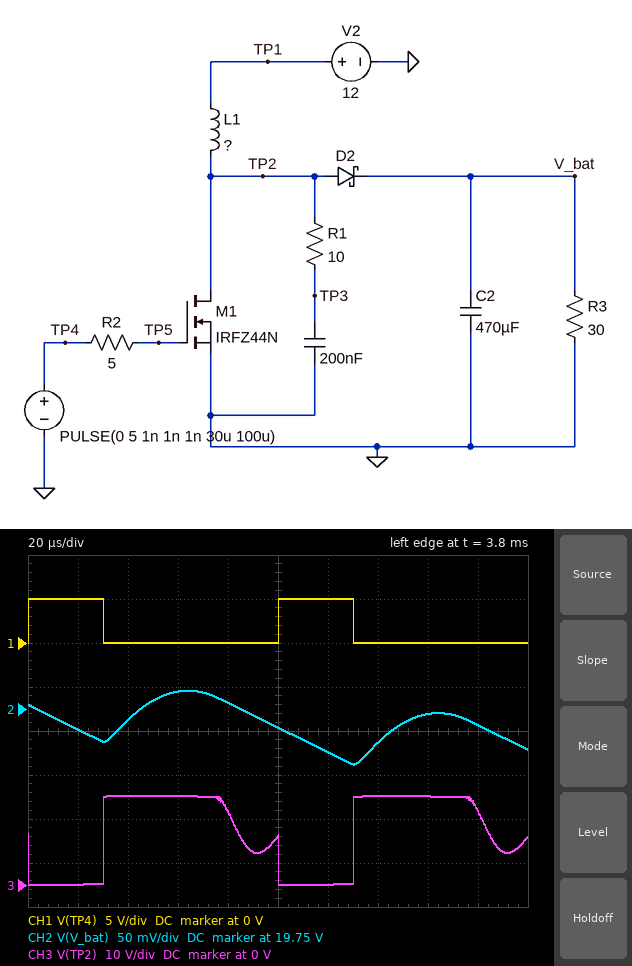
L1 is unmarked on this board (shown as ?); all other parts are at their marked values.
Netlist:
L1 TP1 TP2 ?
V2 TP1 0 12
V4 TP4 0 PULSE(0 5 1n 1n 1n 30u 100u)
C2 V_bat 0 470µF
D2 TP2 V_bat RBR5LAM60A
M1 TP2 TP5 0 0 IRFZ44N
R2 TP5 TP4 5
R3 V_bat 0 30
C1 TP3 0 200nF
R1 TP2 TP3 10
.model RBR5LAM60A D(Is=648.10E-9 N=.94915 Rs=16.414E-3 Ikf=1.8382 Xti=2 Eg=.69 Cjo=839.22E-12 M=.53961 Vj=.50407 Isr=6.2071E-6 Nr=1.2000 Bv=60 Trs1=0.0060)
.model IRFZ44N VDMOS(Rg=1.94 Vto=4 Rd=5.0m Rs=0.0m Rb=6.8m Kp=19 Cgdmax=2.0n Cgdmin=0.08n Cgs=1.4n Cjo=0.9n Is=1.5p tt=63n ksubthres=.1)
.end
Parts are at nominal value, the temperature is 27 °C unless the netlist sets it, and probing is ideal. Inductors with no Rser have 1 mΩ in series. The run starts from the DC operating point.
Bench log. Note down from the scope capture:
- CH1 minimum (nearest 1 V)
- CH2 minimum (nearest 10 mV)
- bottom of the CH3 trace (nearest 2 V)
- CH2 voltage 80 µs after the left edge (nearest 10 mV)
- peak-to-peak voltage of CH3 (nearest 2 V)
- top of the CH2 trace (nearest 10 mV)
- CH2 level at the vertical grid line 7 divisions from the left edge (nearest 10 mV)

0 V
19.69 V
0 V
19.76 V
20 V
19.77 V
19.71 V
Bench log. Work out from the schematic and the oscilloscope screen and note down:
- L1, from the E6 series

150 µH
